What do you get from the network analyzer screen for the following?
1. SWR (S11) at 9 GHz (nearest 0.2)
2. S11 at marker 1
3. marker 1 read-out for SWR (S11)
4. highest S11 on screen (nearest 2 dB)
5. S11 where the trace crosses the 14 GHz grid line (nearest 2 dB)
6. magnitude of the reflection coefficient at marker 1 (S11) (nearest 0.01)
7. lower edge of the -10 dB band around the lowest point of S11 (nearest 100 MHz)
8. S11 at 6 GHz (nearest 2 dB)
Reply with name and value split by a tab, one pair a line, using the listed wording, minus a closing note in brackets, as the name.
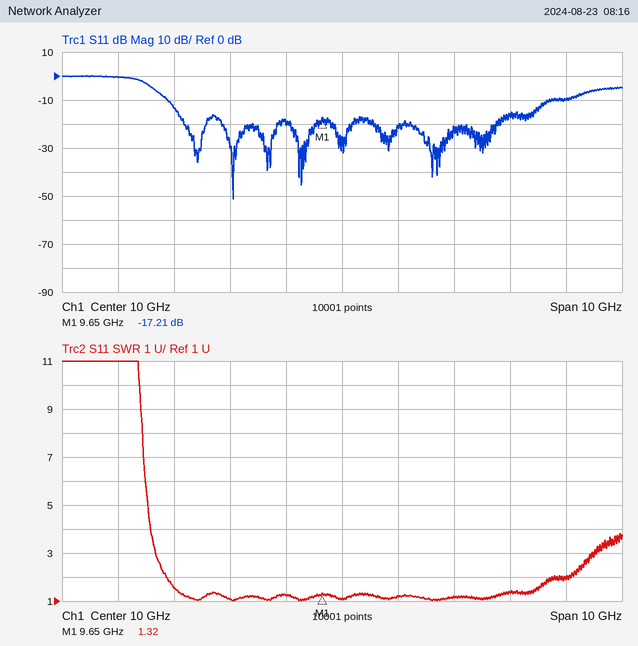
SWR (S11) at 9 GHz	1.2
S11 at marker 1	-17.21 dB
marker 1 read-out for SWR	1.32
highest S11 on screen	0 dB
S11 where the trace crosses the 14 GHz grid line	-10 dB
magnitude of the reflection coefficient at marker 1 (S11)	0.14
lower edge of the -10 dB band around the lowest point of S11	6.9 GHz
S11 at 6 GHz	0 dB
